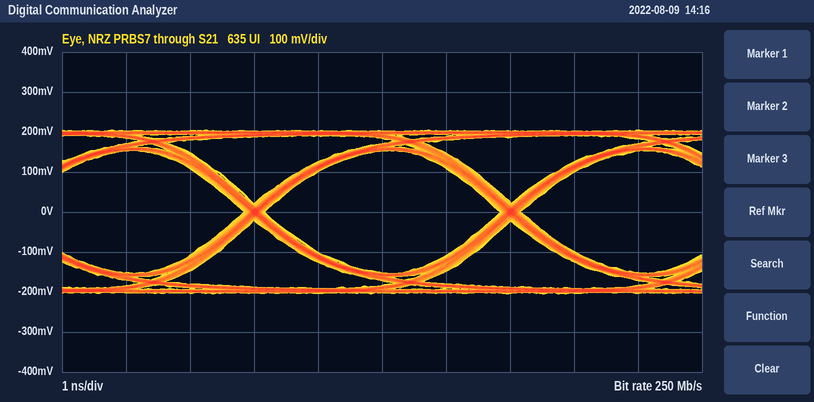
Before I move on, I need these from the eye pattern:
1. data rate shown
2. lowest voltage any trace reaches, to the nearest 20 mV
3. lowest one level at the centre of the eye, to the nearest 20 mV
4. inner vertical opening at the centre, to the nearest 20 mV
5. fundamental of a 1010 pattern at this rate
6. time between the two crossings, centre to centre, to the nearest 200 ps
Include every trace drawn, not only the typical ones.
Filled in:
250 Mb/s
-200 mV
160 mV
300 mV
125 MHz
4.0 ns
